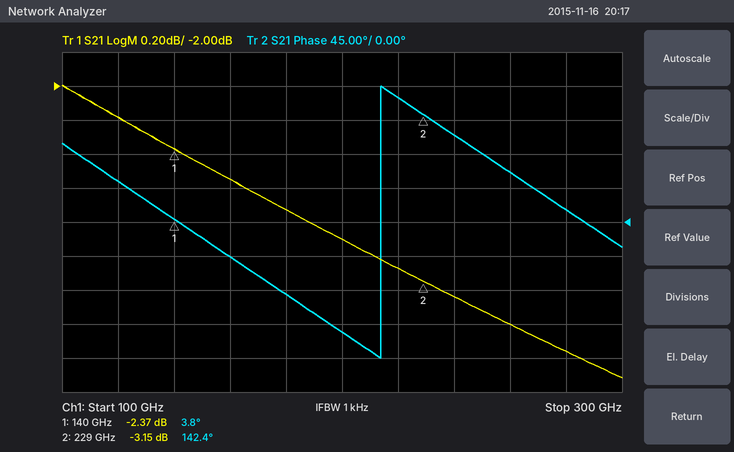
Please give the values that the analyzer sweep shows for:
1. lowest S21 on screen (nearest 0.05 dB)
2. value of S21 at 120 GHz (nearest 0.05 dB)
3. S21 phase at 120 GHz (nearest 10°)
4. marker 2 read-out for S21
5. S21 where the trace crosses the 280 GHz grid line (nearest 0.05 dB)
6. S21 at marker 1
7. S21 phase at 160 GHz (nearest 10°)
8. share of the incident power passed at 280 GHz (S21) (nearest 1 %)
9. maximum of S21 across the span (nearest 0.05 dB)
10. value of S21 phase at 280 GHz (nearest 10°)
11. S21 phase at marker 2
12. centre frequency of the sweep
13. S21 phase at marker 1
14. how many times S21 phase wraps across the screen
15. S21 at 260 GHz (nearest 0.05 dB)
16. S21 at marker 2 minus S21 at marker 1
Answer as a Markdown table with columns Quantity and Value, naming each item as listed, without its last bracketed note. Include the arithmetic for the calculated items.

| Quantity | Value |
|---|---|
| lowest S21 on screen | -3.70 dB |
| value of S21 at 120 GHz | -2.20 dB |
| S21 phase at 120 GHz | 50° |
| marker 2 read-out for S21 | -3.15 dB |
| S21 where the trace crosses the 280 GHz grid line | -3.55 dB |
| S21 at marker 1 | -2.37 dB |
| S21 phase at 160 GHz | -50° |
| share of the incident power passed at 280 GHz (S21) | 10^(-3.55/10) ≈ 44 % |
| maximum of S21 across the span | -2.00 dB |
| value of S21 phase at 280 GHz | 20° |
| S21 phase at marker 2 | 142.4° |
| centre frequency of the sweep | 200 GHz |
| S21 phase at marker 1 | 3.8° |
| how many times S21 phase wraps across the screen | 1 |
| S21 at 260 GHz | -3.40 dB |
| S21 at marker 2 minus S21 at marker 1 | -3.15 − (-2.37) = -0.78 dB |
